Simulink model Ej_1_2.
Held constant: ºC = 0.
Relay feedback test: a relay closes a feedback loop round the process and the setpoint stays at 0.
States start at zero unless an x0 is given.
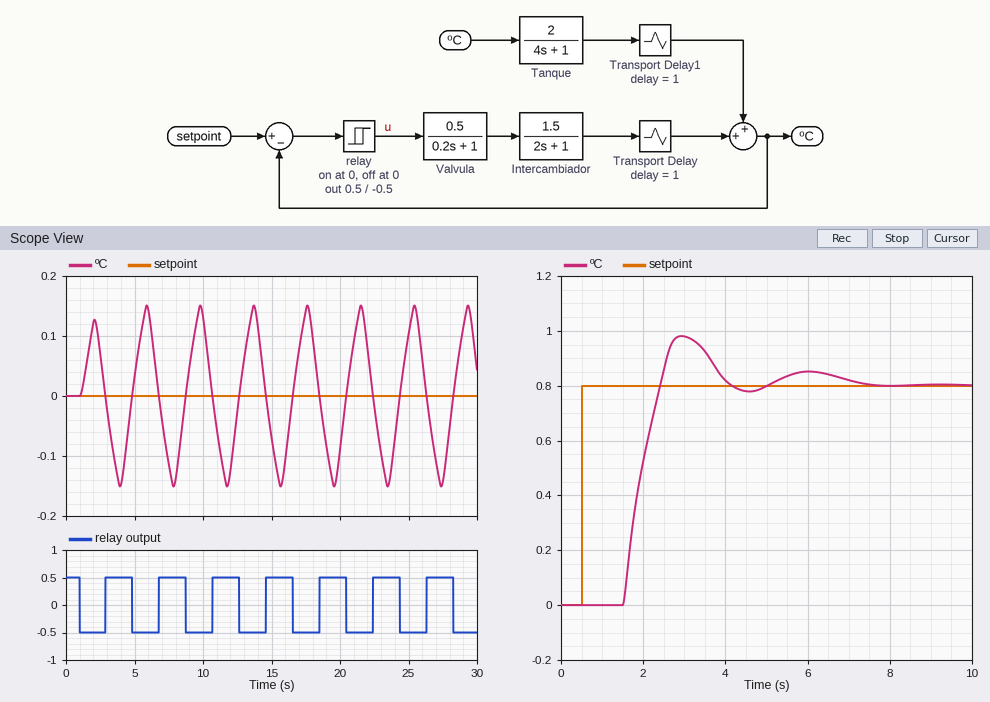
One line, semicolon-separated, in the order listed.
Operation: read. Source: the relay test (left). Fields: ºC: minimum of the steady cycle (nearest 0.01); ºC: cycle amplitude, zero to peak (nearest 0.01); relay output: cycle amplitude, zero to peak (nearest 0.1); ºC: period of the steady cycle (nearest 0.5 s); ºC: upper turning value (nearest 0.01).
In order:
-0.15; 0.15; 0.5; 4.0 s; 0.15
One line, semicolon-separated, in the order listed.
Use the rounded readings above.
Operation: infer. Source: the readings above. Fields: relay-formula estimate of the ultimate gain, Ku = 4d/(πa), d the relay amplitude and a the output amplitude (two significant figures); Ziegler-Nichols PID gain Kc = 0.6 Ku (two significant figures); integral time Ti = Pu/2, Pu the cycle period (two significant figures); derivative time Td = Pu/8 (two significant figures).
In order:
4.2; 2.5; 2.0 s; 0.50 s
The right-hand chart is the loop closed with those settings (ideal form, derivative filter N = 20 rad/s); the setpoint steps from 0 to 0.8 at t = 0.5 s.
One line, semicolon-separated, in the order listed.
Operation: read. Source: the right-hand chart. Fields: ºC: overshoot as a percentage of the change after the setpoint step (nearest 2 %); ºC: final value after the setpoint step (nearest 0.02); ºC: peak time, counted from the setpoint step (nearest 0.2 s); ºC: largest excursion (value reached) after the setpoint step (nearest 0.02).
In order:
22 %; 0.80; 2.4 s; 0.98
